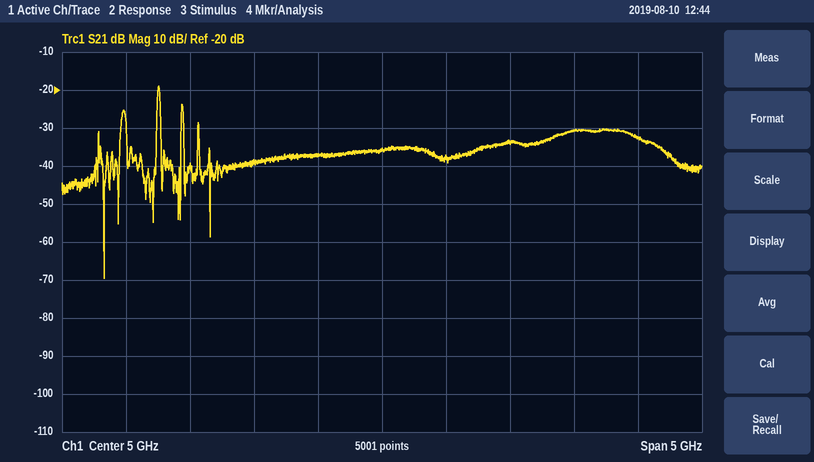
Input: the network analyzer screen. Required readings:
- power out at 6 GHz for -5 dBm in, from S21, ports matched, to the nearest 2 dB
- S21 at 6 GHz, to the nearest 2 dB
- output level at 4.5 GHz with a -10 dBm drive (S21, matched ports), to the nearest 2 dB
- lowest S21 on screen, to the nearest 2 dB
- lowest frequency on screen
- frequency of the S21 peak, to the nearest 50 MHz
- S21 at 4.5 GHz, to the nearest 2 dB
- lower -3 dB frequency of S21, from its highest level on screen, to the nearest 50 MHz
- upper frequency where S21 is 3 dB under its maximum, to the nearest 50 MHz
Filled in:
-38 dBm
-34 dB
-48 dBm
-70 dB
2.5 GHz
3.25 GHz
-38 dB
3.25 GHz
3.25 GHz
